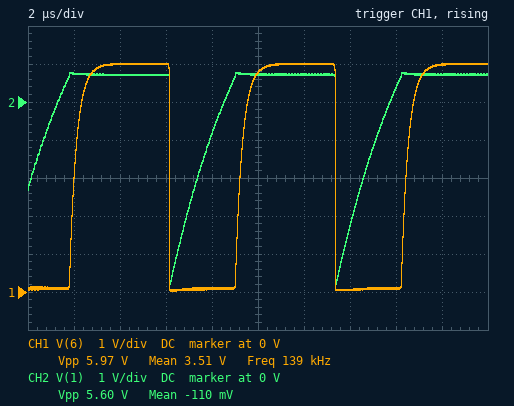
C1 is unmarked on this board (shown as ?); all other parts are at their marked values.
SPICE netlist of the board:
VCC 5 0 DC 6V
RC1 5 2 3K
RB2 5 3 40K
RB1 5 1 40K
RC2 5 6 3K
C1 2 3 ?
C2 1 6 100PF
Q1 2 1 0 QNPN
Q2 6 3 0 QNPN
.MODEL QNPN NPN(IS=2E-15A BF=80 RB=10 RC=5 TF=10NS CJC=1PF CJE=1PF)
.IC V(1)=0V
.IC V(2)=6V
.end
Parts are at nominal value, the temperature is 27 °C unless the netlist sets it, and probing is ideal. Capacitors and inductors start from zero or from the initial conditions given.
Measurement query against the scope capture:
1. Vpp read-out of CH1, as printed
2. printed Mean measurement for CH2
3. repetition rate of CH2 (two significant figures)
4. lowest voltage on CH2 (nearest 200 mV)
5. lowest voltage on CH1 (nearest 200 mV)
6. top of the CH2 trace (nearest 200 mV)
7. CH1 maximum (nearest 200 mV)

5.97 V
-110 mV
140 kHz
-4.8 V
0 V
800 mV
6.0 V
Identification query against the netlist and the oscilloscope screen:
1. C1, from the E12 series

150 pF
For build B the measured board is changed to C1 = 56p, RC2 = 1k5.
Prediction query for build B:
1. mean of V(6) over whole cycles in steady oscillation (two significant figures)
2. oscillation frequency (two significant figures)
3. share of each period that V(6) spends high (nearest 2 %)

2.0 V
230 kHz
32 %
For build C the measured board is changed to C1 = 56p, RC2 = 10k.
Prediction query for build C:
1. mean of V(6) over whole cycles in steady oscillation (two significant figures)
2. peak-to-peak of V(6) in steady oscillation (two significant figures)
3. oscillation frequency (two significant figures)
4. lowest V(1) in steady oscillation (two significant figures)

1.3 V
4.8 V
240 kHz
-3.7 V
